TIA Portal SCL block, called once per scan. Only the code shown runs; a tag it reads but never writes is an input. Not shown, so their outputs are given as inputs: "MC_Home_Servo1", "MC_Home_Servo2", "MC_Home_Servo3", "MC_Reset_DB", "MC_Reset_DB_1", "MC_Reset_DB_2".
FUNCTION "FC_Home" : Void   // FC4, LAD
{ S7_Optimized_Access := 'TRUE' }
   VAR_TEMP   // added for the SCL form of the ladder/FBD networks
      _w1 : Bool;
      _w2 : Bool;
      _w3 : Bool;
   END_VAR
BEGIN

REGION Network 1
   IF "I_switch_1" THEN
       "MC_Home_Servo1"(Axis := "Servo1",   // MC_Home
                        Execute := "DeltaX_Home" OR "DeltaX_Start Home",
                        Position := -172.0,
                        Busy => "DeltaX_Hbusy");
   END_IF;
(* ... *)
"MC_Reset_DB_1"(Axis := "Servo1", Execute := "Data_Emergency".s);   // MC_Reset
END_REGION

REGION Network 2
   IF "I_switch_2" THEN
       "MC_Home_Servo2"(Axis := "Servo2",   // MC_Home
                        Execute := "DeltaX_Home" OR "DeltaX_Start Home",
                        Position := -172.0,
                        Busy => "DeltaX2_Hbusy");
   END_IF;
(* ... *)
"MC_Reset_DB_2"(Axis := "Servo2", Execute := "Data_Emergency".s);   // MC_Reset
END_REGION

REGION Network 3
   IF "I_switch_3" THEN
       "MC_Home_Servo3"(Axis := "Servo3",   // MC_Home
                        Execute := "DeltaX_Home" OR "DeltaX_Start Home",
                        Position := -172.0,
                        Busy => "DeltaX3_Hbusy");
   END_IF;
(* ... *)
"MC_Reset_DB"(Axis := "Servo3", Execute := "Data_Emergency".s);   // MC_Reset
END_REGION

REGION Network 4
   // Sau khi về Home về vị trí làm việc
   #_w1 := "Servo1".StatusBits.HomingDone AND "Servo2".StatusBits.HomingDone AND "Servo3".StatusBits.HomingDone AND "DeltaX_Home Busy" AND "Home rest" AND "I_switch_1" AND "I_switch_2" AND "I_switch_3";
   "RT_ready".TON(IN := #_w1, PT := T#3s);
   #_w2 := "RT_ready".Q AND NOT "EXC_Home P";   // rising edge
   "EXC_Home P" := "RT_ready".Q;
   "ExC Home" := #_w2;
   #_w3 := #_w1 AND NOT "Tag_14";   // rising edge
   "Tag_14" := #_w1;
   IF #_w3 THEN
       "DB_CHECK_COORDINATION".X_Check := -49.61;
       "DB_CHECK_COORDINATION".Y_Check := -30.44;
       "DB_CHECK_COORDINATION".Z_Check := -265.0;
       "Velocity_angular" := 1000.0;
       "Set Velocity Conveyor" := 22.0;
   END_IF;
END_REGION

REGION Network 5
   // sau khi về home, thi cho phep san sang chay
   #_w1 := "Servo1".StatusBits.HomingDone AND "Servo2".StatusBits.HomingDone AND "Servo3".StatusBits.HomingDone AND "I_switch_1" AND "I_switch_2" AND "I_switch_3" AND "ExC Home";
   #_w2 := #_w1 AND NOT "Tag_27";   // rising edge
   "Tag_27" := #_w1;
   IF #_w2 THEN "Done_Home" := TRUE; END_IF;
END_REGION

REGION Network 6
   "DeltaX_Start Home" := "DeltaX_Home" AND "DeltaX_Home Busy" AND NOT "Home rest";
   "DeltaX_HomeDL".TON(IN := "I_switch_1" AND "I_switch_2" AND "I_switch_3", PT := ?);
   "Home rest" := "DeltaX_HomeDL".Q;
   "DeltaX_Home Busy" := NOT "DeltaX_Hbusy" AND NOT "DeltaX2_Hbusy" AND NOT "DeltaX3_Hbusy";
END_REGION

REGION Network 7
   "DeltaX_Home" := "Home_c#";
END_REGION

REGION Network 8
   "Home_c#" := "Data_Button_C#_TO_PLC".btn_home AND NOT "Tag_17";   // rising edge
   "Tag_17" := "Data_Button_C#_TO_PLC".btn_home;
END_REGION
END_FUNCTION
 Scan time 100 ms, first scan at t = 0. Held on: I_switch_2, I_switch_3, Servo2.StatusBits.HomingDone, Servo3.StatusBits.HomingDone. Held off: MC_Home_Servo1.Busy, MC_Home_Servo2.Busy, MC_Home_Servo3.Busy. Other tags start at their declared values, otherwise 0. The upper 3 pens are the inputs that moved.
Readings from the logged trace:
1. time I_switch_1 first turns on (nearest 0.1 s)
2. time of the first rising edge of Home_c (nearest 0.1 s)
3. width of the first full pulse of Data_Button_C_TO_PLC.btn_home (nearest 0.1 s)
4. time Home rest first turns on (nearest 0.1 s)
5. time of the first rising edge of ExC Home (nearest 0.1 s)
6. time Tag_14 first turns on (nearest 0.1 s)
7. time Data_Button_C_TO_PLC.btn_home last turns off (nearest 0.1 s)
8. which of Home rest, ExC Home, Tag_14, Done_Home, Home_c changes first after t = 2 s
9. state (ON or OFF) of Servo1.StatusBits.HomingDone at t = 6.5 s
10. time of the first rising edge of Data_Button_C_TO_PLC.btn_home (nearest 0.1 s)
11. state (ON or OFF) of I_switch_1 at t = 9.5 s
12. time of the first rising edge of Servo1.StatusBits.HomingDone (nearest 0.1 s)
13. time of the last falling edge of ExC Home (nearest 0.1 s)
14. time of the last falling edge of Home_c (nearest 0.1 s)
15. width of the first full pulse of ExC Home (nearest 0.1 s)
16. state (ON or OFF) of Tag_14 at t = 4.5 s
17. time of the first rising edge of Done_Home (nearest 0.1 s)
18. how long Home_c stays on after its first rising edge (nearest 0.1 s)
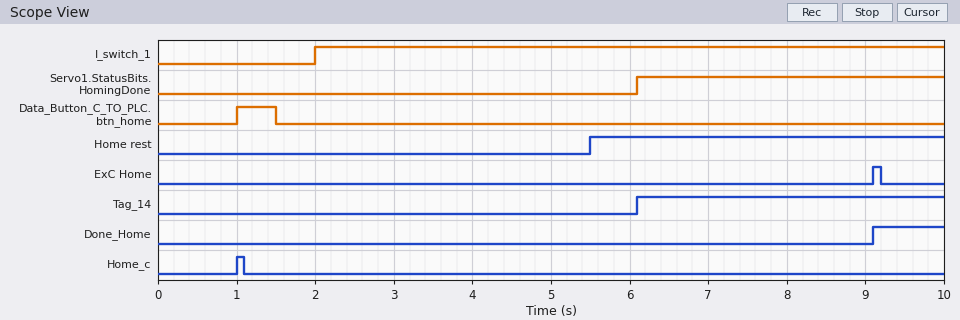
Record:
2.0 s
1.0 s
0.5 s
5.5 s
9.1 s
6.1 s
1.5 s
Home rest
ON
1.0 s
ON
6.1 s
9.2 s
1.1 s
0.1 s
OFF
9.1 s
0.1 s
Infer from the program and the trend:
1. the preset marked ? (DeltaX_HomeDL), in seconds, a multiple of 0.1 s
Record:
3.5 s
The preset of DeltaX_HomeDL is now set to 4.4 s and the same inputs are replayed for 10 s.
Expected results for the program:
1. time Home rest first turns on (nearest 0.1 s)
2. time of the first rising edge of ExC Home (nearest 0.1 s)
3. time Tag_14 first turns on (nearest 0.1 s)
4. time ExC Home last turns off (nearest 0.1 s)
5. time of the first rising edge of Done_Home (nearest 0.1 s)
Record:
6.4 s
9.5 s
6.5 s
9.6 s
9.5 s
